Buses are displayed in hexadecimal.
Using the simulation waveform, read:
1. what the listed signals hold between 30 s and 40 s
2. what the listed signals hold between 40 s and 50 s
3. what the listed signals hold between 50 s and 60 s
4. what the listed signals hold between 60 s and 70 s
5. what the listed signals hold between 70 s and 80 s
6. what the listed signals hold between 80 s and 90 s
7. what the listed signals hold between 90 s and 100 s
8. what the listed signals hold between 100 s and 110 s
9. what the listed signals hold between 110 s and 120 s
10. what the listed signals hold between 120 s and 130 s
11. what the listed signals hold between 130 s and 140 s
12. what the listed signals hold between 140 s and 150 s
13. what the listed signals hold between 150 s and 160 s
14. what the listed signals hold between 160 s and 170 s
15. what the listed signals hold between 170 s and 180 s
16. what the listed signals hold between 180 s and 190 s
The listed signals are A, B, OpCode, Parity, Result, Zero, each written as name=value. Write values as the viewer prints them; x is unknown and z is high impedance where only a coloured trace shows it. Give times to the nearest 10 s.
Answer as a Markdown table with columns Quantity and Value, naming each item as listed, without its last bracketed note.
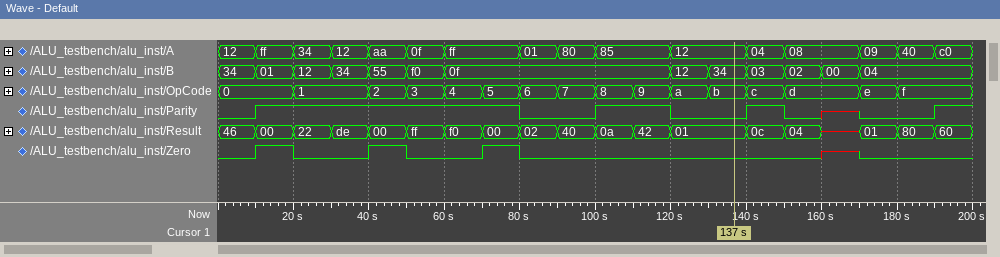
| Quantity | Value |
|---|---|
| what the listed signals hold between 30 s and 40 s | A=12, B=34, OpCode=1, Parity=1, Result=de, Zero=0 |
| what the listed signals hold between 40 s and 50 s | A=aa, B=55, OpCode=2, Parity=1, Result=00, Zero=1 |
| what the listed signals hold between 50 s and 60 s | A=0f, B=f0, OpCode=3, Parity=1, Result=ff, Zero=0 |
| what the listed signals hold between 60 s and 70 s | A=ff, B=0f, OpCode=4, Parity=1, Result=f0, Zero=0 |
| what the listed signals hold between 70 s and 80 s | A=ff, B=0f, OpCode=5, Parity=1, Result=00, Zero=1 |
| what the listed signals hold between 80 s and 90 s | A=01, B=0f, OpCode=6, Parity=0, Result=02, Zero=0 |
| what the listed signals hold between 90 s and 100 s | A=80, B=0f, OpCode=7, Parity=0, Result=40, Zero=0 |
| what the listed signals hold between 100 s and 110 s | A=85, B=0f, OpCode=8, Parity=1, Result=0a, Zero=0 |
| what the listed signals hold between 110 s and 120 s | A=85, B=0f, OpCode=9, Parity=1, Result=42, Zero=0 |
| what the listed signals hold between 120 s and 130 s | A=12, B=12, OpCode=a, Parity=0, Result=01, Zero=0 |
| what the listed signals hold between 130 s and 140 s | A=12, B=34, OpCode=b, Parity=0, Result=01, Zero=0 |
| what the listed signals hold between 140 s and 150 s | A=04, B=03, OpCode=c, Parity=1, Result=0c, Zero=0 |
| what the listed signals hold between 150 s and 160 s | A=08, B=02, OpCode=d, Parity=0, Result=04, Zero=0 |
| what the listed signals hold between 160 s and 170 s | A=08, B=00, OpCode=d, Parity=x, Result=x, Zero=x |
| what the listed signals hold between 170 s and 180 s | A=09, B=04, OpCode=e, Parity=0, Result=01, Zero=0 |
| what the listed signals hold between 180 s and 190 s | A=40, B=04, OpCode=f, Parity=0, Result=80, Zero=0 |
